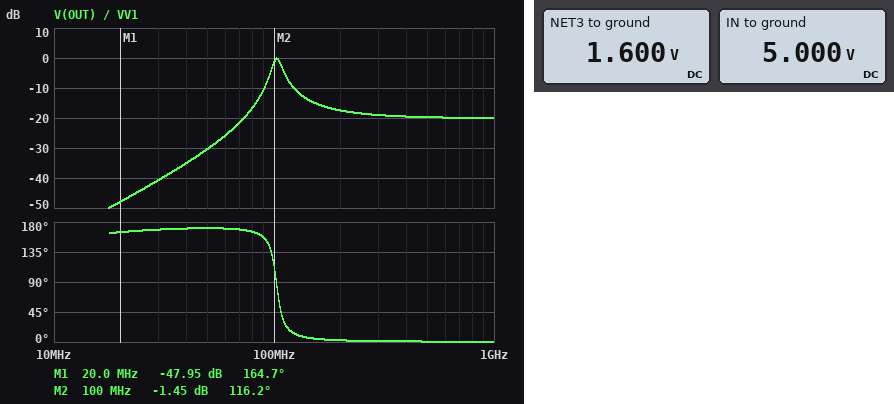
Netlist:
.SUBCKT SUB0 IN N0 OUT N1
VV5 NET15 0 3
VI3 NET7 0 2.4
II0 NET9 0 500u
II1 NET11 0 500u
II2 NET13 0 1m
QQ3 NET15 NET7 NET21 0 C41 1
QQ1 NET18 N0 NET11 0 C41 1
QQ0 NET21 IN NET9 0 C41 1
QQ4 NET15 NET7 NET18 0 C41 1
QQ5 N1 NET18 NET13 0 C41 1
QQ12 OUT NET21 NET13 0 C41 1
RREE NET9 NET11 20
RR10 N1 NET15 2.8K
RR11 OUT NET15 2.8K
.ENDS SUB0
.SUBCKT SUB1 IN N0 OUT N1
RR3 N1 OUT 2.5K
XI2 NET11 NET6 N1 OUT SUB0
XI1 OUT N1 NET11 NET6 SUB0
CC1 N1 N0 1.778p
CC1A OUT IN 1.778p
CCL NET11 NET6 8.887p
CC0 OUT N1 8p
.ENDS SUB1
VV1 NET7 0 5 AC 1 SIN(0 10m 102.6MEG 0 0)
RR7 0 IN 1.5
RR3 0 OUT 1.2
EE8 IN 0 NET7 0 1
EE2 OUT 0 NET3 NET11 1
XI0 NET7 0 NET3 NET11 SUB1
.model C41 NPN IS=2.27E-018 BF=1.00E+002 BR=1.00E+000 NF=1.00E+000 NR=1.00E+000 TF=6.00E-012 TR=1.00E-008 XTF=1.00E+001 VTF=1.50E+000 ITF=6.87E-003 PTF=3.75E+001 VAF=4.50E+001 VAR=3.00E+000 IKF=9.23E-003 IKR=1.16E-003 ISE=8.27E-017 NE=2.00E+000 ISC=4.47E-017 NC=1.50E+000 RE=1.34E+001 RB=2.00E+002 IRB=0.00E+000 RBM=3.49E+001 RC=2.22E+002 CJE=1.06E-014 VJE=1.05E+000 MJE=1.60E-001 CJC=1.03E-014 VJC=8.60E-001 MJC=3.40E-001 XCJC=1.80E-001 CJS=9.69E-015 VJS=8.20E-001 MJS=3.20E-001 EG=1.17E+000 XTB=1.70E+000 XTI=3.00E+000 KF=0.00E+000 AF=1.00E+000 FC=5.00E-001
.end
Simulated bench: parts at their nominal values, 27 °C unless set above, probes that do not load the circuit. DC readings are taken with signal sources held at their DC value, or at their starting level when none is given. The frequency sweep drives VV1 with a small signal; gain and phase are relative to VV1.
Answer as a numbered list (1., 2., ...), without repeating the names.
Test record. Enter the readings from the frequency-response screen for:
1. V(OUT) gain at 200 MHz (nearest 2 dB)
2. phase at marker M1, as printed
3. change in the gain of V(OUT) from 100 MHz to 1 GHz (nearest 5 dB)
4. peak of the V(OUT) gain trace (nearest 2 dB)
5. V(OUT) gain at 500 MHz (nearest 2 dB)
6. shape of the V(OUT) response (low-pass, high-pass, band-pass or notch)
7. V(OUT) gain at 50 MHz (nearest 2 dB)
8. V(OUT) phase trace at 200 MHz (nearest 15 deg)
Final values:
1. -18 dB
2. 164.7 deg
3. -20 dB
4. 0 dB
5. -20 dB
6. high-pass
7. -30 dB
8. 0 deg
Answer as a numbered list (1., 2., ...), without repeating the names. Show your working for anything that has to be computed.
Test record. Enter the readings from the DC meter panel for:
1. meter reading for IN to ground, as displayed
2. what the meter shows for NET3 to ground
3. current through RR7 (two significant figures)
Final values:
1. 5.000 V
2. 1.600 V
3. (5 V) / 1.5 Ω = 3.3 A
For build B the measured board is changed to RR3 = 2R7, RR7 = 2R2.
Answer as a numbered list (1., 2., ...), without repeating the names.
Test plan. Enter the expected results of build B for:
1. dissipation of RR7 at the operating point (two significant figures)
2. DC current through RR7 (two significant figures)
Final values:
1. 11 W
2. 2.3 A
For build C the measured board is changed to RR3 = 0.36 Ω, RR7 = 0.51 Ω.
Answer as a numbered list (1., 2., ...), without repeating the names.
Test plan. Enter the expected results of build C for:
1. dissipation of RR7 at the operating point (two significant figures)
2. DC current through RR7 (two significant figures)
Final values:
1. 49 W
2. 9.8 A
